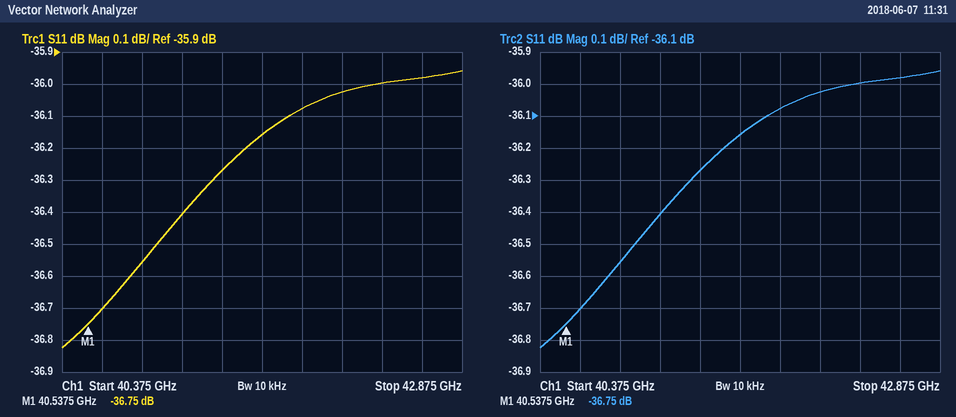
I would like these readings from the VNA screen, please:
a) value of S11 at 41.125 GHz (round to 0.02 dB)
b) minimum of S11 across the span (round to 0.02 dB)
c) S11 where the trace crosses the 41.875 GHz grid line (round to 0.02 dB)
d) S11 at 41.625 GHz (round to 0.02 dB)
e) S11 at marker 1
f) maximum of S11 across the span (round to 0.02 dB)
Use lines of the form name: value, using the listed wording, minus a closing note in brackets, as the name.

value of S11 at 41.125 GHz: -36.40 dB
minimum of S11 across the span: -36.82 dB
S11 where the trace crosses the 41.875 GHz grid line: -36.08 dB
S11 at 41.625 GHz: -36.16 dB
S11 at marker 1: -36.75 dB
maximum of S11 across the span: -35.96 dB
